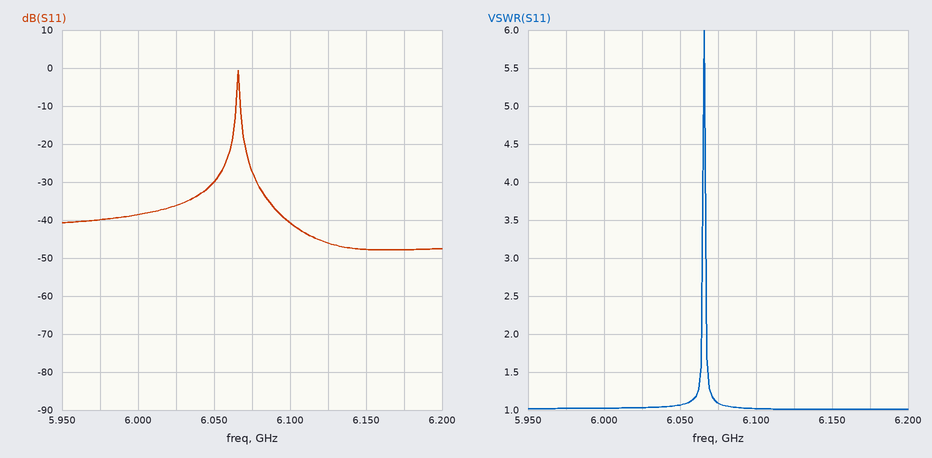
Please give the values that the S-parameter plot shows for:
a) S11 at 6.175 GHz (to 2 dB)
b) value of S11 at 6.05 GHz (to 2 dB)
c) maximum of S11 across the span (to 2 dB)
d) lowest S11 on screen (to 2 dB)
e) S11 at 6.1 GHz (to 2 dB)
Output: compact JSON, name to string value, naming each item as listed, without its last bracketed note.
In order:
{"S11 at 6.175 GHz": "-48 dB", "value of S11 at 6.05 GHz": "-30 dB", "maximum of S11 across the span": "0 dB", "lowest S11 on screen": "-48 dB", "S11 at 6.1 GHz": "-40 dB"}
